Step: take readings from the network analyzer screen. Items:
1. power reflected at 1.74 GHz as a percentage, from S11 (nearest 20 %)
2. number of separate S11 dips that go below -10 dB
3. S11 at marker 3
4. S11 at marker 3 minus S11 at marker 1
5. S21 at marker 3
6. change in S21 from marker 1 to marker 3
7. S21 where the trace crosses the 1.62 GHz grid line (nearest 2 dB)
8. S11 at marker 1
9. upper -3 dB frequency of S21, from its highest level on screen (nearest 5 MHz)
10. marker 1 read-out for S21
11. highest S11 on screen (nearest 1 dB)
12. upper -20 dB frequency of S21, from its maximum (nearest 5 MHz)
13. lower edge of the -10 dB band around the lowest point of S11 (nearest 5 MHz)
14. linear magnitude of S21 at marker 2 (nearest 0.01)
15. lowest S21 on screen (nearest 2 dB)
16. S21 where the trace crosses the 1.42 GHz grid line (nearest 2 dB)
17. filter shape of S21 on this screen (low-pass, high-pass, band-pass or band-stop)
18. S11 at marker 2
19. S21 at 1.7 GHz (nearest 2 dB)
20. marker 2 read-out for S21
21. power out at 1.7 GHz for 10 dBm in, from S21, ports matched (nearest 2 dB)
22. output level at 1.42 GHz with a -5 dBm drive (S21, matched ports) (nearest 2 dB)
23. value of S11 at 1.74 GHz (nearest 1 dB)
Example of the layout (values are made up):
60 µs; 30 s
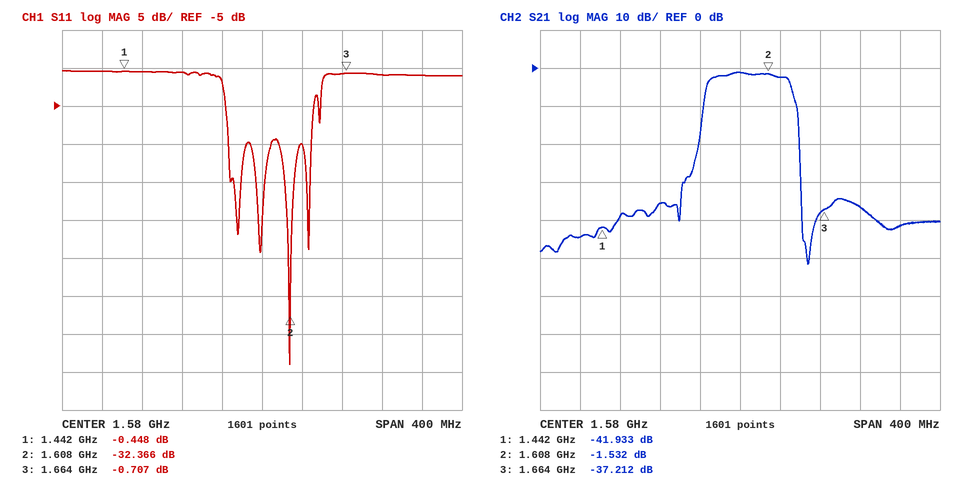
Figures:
80 %; 4; -0.707 dB; -0.259 dB; -37.212 dB; 4.721 dB; -2 dB; -0.448 dB; 1.630 GHz; -41.933 dB; 0 dB; 1.640 GHz; 1.595 GHz; 0.84; -52 dB; -44 dB; band-pass; -32.366 dB; -36 dB; -1.532 dB; -26 dBm; -50 dBm; -1 dB
